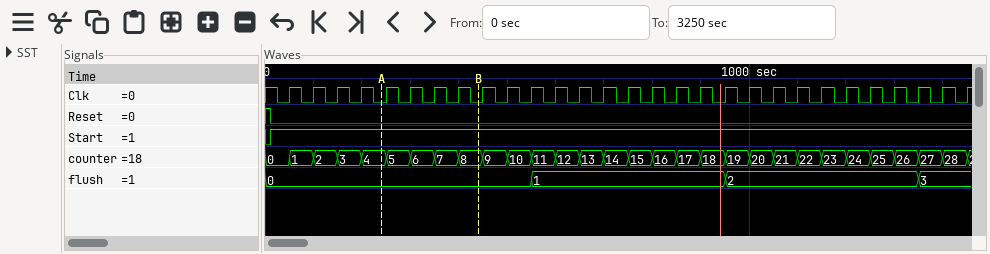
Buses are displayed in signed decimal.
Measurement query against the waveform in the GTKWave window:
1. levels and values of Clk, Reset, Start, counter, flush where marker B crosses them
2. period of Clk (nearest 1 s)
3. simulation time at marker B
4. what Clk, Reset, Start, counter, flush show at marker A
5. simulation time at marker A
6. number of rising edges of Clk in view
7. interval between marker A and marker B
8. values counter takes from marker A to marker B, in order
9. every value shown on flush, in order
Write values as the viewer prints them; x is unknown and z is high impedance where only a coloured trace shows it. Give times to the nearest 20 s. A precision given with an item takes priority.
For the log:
Clk=0, Reset=0, Start=1, counter=8, flush=0
50 s
440 s
Clk=0, Reset=0, Start=1, counter=4, flush=0
240 s
29
200 s
4, 5, 6, 7, 8
0, 1, 2, 3
